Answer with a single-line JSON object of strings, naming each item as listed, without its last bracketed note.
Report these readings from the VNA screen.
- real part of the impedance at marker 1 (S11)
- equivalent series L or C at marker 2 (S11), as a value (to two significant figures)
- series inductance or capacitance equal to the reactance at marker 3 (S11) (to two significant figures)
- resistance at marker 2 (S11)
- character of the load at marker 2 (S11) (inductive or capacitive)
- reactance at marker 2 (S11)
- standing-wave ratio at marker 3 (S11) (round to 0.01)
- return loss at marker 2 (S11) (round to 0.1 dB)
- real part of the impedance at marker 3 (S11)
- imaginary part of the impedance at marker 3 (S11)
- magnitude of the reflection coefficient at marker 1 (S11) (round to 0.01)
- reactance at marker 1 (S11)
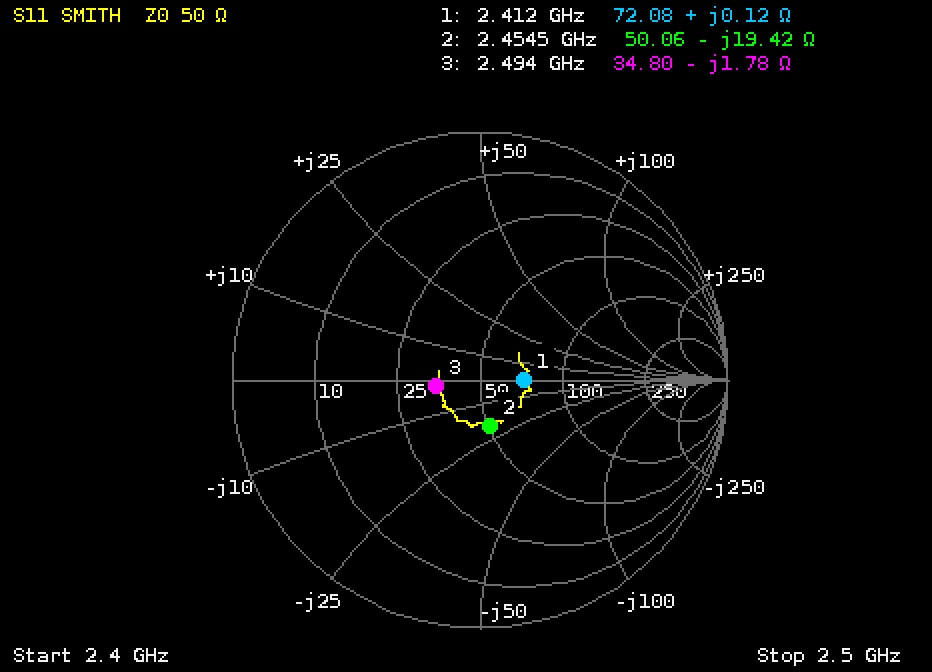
{"real part of the impedance at marker 1": "72.08 Ω", "equivalent series L or C at marker 2 (S11), as a value": "3.3 pF", "series inductance or capacitance equal to the reactance at marker 3 (S11)": "36 pF", "resistance at marker 2": "50.06 Ω", "character of the load at marker 2 (S11)": "capacitive", "reactance at marker 2": "-19.42 Ω", "standing-wave ratio at marker 3 (S11)": "1.44", "return loss at marker 2 (S11)": "14.4 dB", "real part of the impedance at marker 3": "34.80 Ω", "imaginary part of the impedance at marker 3": "-1.78 Ω", "magnitude of the reflection coefficient at marker 1 (S11)": "0.18", "reactance at marker 1": "+0.12 Ω"}
